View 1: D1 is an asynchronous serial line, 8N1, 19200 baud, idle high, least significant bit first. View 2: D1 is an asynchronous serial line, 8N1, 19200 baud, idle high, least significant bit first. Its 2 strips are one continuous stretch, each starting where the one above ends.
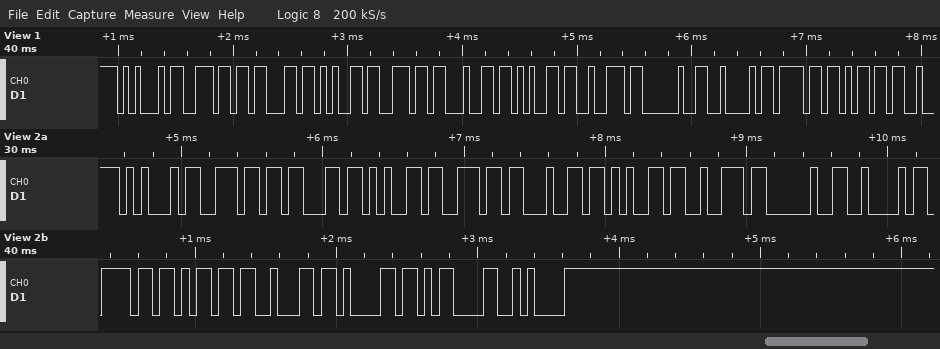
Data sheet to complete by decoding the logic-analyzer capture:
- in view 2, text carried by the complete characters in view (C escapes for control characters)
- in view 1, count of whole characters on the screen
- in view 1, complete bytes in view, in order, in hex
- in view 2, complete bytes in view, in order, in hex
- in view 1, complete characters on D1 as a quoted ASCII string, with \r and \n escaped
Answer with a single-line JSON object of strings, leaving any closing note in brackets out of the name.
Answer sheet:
{"in view 2, text carried by the complete characters in view": "\"Encender Bomba\\r\\n\"", "in view 1, count of whole characters on the screen": "12", "in view 1, complete bytes in view, in order, in hex": "45 6E 63 65 6E 64 65 72 20 42 6F 6D", "in view 2, complete bytes in view, in order, in hex": "45 6E 63 65 6E 64 65 72 20 42 6F 6D 62 61 0D 0A", "in view 1, complete characters on D1 as a quoted ASCII string, with \\r and \\n escaped": "\"Encender Bom\""}
